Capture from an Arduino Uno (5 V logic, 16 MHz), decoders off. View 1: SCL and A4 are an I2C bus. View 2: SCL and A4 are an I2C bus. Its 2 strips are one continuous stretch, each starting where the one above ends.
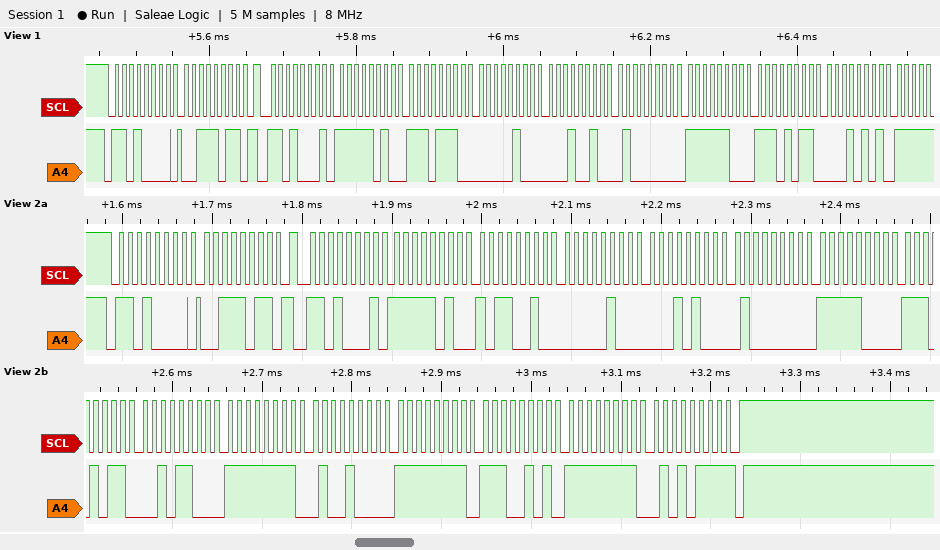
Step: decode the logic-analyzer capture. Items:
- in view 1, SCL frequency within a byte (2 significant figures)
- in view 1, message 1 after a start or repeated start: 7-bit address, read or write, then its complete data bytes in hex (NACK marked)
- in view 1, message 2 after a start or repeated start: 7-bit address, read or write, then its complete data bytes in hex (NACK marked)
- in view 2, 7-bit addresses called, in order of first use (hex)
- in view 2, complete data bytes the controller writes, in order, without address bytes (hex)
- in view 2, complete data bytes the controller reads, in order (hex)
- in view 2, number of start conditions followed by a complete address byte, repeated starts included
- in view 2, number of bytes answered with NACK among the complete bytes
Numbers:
100 kHz
0x68 write: 3B
0x68 read: FA EE 04 12 40 FC EB 15
0x68
3B
FA B2 04 14 40 F8 EB 2C FF 48 FF E5 FF 57
2
1
